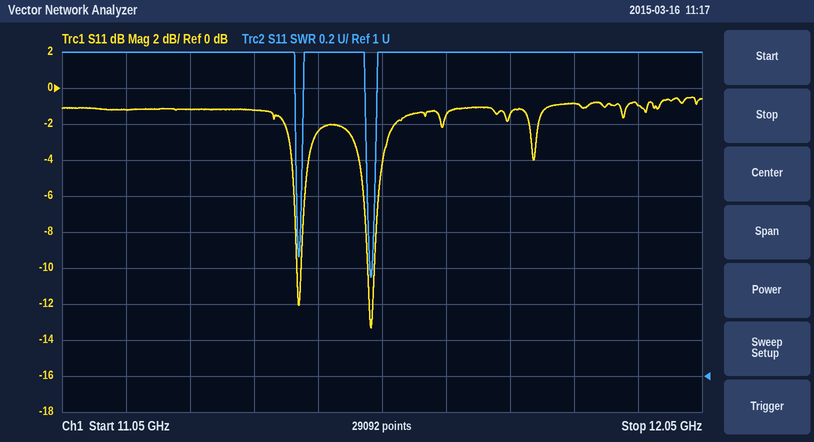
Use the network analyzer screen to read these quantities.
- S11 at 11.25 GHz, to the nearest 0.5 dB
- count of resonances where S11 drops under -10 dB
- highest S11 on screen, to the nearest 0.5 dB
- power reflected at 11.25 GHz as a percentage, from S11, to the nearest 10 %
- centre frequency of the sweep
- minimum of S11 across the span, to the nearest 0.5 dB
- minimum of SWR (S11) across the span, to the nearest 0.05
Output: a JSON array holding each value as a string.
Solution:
["-1.0 dB", "2", "-0.5 dB", "80 %", "11.55 GHz", "-13.5 dB", "1.55"]
